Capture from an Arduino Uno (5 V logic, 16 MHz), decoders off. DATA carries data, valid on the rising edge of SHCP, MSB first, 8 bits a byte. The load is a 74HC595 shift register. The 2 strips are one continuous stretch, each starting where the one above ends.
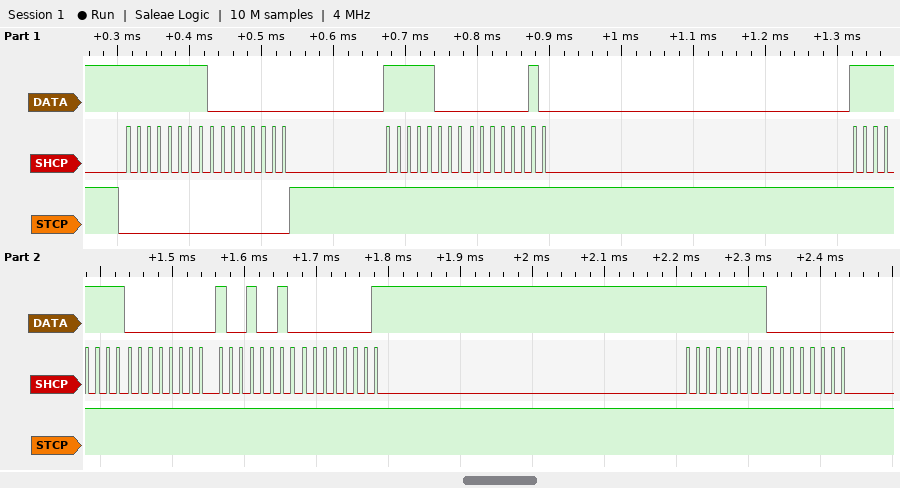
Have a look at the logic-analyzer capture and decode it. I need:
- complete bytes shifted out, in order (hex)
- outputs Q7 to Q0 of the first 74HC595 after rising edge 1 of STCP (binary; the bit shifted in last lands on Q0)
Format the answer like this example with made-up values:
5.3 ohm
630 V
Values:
0xFF 0x00 0xF8 0x02 0xFF 0x00 0x92 0x01 0xFF 0x00
00000000
